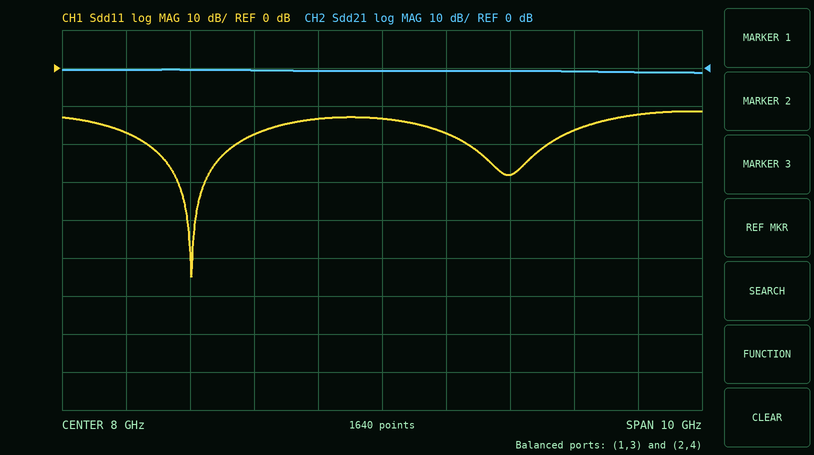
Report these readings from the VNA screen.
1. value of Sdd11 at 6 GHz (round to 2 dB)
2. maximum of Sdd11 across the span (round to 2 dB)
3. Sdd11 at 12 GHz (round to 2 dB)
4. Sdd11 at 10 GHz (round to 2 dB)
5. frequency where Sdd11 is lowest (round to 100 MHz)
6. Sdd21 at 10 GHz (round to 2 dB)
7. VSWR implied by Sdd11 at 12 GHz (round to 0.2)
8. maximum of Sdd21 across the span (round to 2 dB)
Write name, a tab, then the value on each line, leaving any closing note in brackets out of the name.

value of Sdd11 at 6 GHz	-18 dB
maximum of Sdd11 across the span	-12 dB
Sdd11 at 12 GHz	-12 dB
Sdd11 at 10 GHz	-28 dB
frequency where Sdd11 is lowest	5.0 GHz
Sdd21 at 10 GHz	0 dB
VSWR implied by Sdd11 at 12 GHz	1.6
maximum of Sdd21 across the span	0 dB
